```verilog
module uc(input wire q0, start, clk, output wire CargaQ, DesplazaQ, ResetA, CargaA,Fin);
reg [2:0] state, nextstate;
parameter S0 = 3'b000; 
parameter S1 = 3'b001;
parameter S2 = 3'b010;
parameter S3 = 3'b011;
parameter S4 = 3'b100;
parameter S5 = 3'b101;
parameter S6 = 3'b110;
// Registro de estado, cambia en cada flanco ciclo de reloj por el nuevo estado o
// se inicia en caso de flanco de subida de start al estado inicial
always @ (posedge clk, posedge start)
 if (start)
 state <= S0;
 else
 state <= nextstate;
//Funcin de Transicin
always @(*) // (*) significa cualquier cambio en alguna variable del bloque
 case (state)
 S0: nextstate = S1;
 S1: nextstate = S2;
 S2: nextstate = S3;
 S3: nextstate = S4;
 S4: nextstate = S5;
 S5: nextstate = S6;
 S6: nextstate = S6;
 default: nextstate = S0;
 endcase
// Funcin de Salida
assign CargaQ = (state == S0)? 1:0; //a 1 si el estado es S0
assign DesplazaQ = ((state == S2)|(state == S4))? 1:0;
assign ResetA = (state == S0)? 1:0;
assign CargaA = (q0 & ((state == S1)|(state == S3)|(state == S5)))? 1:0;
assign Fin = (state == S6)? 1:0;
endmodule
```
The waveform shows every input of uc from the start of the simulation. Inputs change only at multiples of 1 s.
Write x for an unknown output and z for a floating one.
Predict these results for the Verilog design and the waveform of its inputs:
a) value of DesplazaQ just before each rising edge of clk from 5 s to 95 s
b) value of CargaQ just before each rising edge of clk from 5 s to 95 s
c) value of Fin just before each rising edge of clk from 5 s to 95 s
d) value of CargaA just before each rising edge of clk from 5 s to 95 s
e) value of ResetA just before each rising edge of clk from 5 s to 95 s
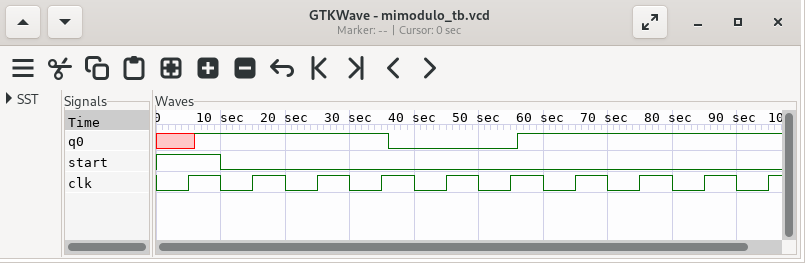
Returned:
0 0 0 1 0 1 0 0 0 0
1 1 0 0 0 0 0 0 0 0
0 0 0 0 0 0 0 1 1 1
0 0 1 0 0 0 1 0 0 0
1 1 0 0 0 0 0 0 0 0
